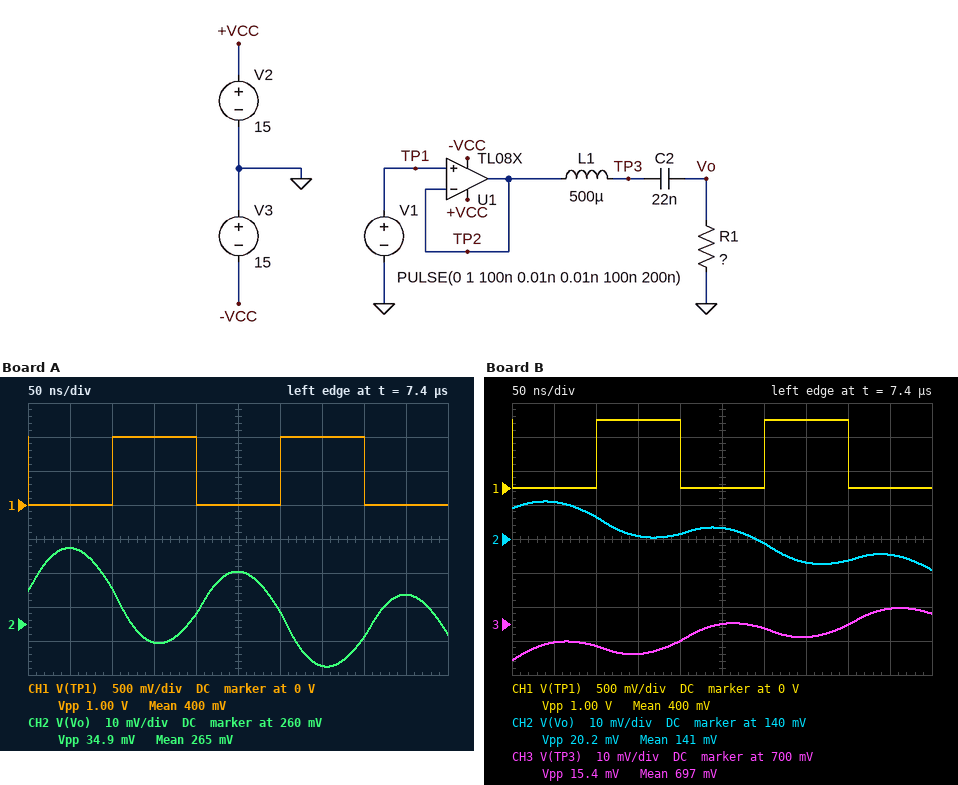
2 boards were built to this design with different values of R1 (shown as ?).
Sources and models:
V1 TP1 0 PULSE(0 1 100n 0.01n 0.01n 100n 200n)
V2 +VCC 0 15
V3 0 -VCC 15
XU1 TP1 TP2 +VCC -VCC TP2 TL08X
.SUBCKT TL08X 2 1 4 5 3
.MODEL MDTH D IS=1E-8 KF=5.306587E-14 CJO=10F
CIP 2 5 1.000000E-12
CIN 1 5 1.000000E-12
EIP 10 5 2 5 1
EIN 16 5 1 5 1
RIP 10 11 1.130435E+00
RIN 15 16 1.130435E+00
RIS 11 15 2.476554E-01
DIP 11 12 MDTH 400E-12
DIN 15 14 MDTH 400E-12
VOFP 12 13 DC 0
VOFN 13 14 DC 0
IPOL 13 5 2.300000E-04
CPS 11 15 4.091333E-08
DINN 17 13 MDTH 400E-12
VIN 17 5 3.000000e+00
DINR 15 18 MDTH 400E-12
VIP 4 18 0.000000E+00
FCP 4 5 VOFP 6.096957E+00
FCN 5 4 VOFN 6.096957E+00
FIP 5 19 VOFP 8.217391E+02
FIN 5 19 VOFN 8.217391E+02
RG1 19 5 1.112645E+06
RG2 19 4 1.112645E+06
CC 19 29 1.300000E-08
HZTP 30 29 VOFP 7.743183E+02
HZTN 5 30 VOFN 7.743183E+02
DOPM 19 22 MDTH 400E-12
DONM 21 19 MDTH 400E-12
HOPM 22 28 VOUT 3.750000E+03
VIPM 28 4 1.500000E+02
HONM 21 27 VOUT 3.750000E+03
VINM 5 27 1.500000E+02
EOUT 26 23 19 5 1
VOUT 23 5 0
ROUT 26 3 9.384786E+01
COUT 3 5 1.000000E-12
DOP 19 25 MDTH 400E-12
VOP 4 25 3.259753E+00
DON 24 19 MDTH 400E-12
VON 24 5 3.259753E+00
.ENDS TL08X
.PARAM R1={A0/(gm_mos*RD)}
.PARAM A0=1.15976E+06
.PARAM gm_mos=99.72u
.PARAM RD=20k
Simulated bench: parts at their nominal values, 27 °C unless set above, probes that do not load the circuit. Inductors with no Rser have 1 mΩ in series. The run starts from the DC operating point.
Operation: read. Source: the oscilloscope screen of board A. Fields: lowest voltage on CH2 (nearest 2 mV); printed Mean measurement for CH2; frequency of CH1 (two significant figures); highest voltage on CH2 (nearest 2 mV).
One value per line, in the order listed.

248 mV
265 mV
5.0 MHz
282 mV
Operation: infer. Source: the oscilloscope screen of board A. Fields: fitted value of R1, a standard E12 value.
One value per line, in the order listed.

390 Ω
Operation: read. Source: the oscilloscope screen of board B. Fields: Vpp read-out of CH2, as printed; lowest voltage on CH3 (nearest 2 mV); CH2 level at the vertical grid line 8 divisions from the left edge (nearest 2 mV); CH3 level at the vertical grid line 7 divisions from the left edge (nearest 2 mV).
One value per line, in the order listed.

20.2 mV
690 mV
134 mV
696 mV
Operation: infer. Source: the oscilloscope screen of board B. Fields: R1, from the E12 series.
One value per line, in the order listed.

100 Ω
